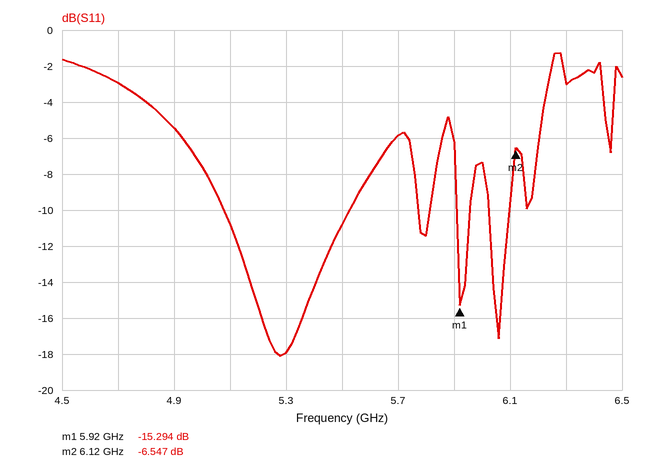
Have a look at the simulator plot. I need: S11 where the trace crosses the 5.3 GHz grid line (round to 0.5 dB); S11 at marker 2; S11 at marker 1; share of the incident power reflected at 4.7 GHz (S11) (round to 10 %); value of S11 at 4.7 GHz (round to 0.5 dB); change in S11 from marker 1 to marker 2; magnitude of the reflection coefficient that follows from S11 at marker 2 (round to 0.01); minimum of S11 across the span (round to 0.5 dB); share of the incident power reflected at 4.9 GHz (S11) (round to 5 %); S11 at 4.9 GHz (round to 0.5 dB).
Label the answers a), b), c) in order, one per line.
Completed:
a) -18.0 dB
b) -6.547 dB
c) -15.294 dB
d) 50 %
e) -3.0 dB
f) 8.747 dB
g) 0.47
h) -18.0 dB
i) 30 %
j) -5.5 dB
